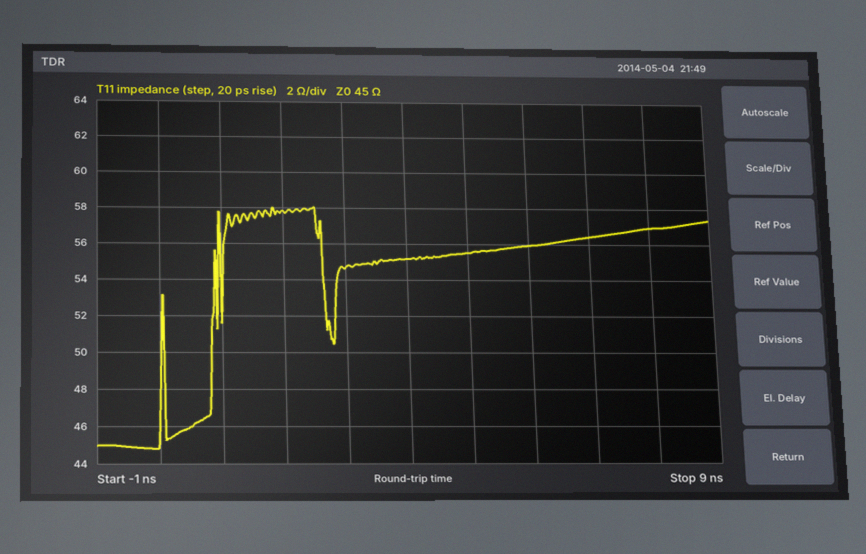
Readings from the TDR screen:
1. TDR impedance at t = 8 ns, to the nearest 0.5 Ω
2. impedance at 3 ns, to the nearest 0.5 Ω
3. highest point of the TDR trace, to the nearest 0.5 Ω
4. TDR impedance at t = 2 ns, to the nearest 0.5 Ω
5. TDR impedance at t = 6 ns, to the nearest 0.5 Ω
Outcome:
57.0 Ω
54.5 Ω
58.0 Ω
58.0 Ω
56.0 Ω
